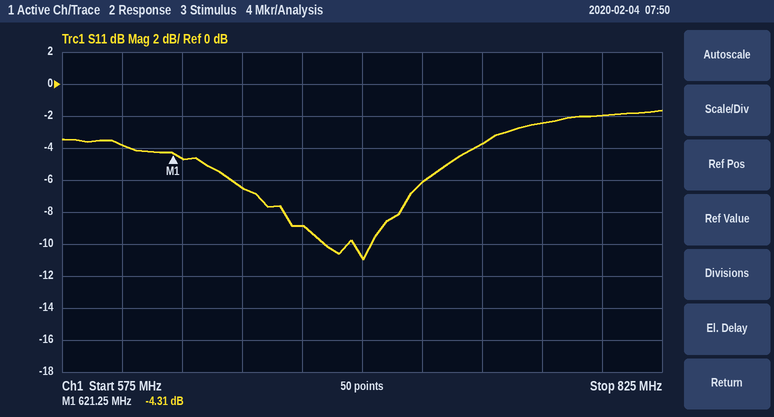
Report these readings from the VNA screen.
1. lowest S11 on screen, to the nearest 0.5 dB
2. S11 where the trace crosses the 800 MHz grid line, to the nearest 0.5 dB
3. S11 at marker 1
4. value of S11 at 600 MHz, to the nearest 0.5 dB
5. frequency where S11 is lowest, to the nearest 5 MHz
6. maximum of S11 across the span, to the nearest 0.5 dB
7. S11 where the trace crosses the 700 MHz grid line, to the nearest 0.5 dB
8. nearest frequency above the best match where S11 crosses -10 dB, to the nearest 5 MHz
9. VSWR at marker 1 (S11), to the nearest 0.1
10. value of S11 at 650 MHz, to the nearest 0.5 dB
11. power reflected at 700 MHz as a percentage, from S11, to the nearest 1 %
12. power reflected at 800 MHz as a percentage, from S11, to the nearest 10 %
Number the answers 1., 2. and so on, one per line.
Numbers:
1. -11.0 dB
2. -2.0 dB
3. -4.31 dB
4. -4.0 dB
5. 700 MHz
6. -1.5 dB
7. -11.0 dB
8. 705 MHz
9. 4.1
10. -6.5 dB
11. 8 %
12. 60 %
